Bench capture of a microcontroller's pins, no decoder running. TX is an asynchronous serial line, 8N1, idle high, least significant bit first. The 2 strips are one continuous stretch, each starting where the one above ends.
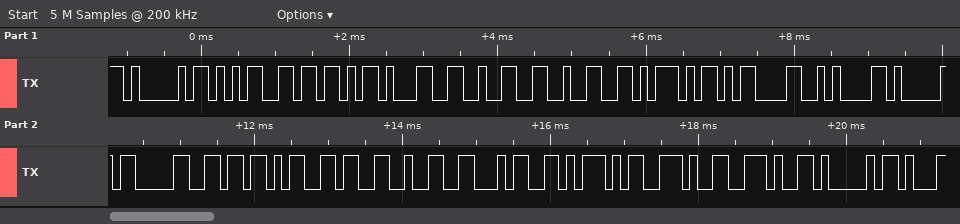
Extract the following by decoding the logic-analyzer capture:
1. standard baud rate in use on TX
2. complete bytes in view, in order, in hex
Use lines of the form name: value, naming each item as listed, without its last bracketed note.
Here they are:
standard baud rate in use on TX: 9600 baud
complete bytes in view, in order, in hex: 41 35 5B 31 32 32 5D 0D 0A 41 30 5B 36 32 34 5D 2E 2E 41
